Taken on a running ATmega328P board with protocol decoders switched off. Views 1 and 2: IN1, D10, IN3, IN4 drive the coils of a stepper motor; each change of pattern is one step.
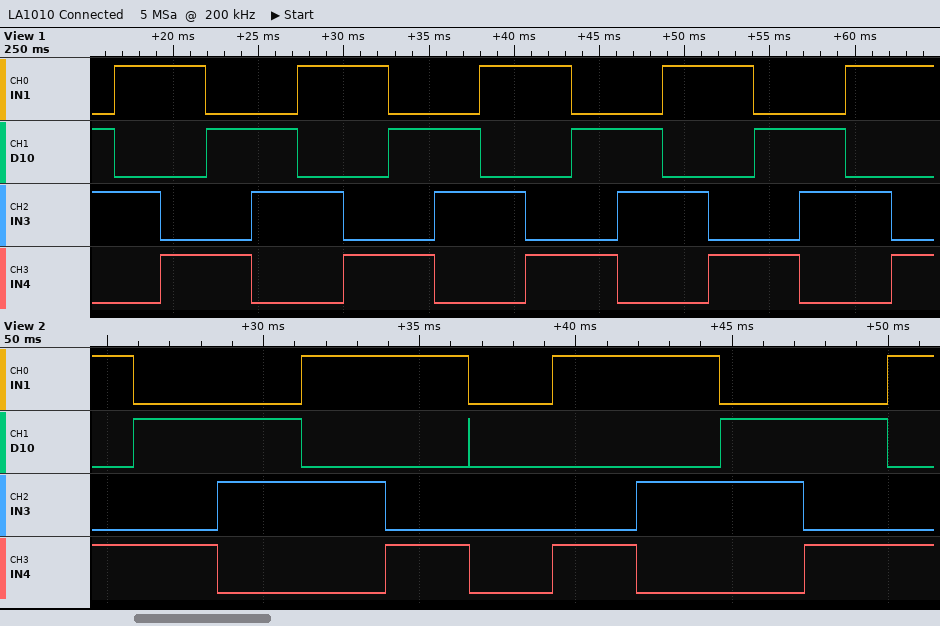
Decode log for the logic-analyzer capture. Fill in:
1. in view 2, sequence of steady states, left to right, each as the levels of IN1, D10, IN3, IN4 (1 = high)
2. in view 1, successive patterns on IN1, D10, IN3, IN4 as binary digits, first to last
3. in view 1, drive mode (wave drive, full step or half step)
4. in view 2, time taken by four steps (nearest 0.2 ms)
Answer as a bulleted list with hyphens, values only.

- 1001 0101 0110 1010 1001 0000 1001 1010 0110 0101 1001
- 0110 1010 1001 0101 0110 1010 1001 0101 0110 1010 1001 0101 0110 1010 1001 0101 0110 1010 1001
- full step
- 10.8 ms
